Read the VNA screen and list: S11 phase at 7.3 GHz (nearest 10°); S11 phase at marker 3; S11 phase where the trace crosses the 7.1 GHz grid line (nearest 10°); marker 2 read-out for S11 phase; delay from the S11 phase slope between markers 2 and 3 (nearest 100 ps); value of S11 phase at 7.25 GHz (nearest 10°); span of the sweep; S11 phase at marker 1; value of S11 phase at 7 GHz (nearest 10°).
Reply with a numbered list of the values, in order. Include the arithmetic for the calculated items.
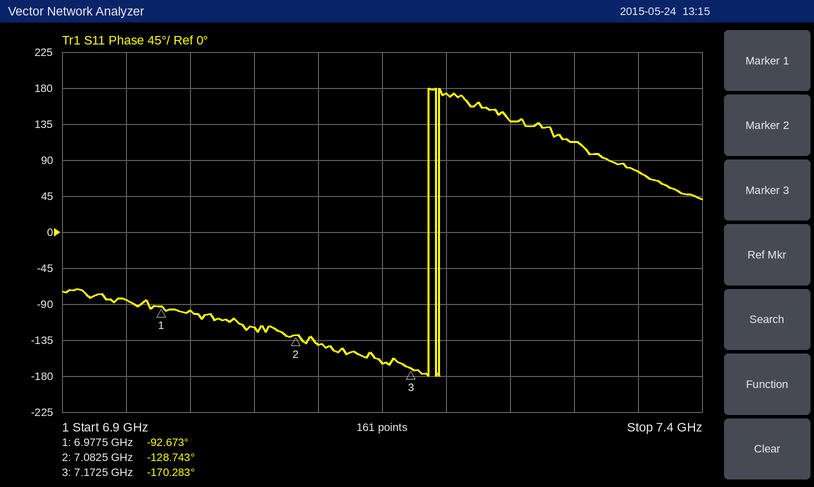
1. 110°
2. -170.283°
3. -140°
4. -128.743°
5. −(-170.283° − (-128.743°))/(360° × 90 MHz) ≈ 1.3 ns
6. 140°
7. 500 MHz
8. -92.673°
9. -100°
